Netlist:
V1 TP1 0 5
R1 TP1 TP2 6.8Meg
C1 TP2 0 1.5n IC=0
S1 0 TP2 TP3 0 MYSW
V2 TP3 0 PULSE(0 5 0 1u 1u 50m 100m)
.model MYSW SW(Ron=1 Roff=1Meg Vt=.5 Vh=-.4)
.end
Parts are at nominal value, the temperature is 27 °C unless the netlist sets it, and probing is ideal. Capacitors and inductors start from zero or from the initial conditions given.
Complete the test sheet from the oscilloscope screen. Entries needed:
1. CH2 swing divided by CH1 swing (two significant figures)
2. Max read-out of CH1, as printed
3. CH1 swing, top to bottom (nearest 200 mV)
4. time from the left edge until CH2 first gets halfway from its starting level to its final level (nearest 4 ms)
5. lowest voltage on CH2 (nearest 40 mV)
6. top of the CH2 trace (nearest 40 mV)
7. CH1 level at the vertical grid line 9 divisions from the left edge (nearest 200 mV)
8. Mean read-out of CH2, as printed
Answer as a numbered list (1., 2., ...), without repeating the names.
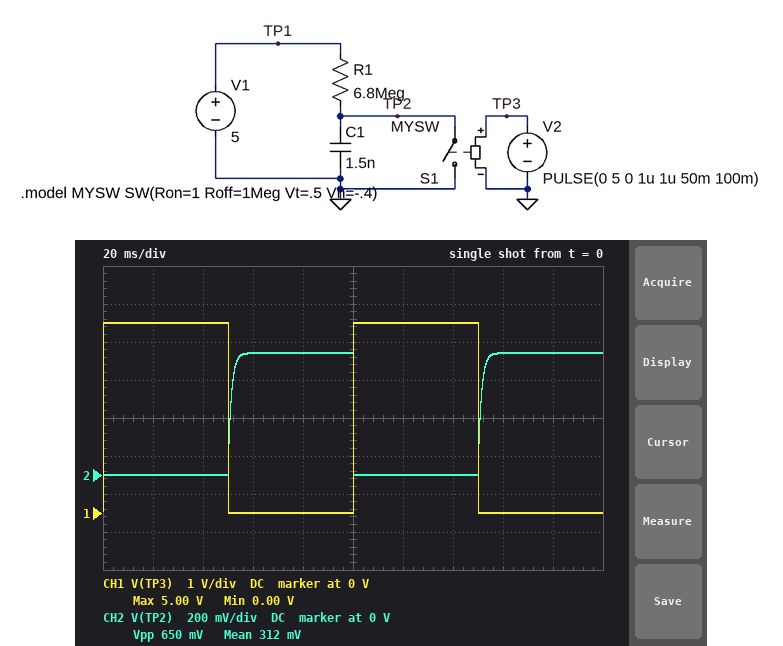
1. 0.13
2. 5.00 V
3. 5.0 V
4. 52 ms
5. 0 V
6. 640 mV
7. 0 V
8. 312 mV
